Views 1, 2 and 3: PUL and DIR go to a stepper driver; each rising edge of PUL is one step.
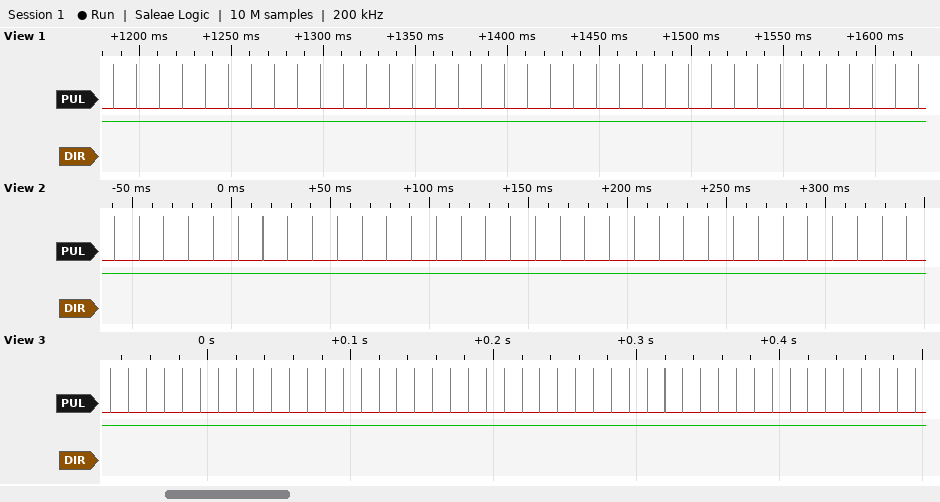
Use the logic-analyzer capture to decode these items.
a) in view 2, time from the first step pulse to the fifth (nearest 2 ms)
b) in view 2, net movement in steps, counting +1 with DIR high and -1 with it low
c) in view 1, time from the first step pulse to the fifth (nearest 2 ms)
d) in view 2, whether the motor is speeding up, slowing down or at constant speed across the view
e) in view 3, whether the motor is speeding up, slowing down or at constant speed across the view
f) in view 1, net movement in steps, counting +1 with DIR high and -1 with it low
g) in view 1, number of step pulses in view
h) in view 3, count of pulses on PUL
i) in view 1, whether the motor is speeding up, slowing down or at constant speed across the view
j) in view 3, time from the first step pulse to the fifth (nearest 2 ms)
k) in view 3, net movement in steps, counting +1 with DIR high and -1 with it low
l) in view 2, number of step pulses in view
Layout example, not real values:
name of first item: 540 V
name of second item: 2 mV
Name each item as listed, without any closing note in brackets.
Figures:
in view 2, time from the first step pulse to the fifth: 50 ms
in view 2, net movement in steps, counting +1 with DIR high and -1 with it low: +33
in view 1, time from the first step pulse to the fifth: 50 ms
in view 2, whether the motor is speeding up, slowing down or at constant speed across the view: constant speed
in view 3, whether the motor is speeding up, slowing down or at constant speed across the view: constant speed
in view 1, net movement in steps, counting +1 with DIR high and -1 with it low: +36
in view 1, number of step pulses in view: 36
in view 3, count of pulses on PUL: 46
in view 1, whether the motor is speeding up, slowing down or at constant speed across the view: constant speed
in view 3, time from the first step pulse to the fifth: 50 ms
in view 3, net movement in steps, counting +1 with DIR high and -1 with it low: +46
in view 2, number of step pulses in view: 33
